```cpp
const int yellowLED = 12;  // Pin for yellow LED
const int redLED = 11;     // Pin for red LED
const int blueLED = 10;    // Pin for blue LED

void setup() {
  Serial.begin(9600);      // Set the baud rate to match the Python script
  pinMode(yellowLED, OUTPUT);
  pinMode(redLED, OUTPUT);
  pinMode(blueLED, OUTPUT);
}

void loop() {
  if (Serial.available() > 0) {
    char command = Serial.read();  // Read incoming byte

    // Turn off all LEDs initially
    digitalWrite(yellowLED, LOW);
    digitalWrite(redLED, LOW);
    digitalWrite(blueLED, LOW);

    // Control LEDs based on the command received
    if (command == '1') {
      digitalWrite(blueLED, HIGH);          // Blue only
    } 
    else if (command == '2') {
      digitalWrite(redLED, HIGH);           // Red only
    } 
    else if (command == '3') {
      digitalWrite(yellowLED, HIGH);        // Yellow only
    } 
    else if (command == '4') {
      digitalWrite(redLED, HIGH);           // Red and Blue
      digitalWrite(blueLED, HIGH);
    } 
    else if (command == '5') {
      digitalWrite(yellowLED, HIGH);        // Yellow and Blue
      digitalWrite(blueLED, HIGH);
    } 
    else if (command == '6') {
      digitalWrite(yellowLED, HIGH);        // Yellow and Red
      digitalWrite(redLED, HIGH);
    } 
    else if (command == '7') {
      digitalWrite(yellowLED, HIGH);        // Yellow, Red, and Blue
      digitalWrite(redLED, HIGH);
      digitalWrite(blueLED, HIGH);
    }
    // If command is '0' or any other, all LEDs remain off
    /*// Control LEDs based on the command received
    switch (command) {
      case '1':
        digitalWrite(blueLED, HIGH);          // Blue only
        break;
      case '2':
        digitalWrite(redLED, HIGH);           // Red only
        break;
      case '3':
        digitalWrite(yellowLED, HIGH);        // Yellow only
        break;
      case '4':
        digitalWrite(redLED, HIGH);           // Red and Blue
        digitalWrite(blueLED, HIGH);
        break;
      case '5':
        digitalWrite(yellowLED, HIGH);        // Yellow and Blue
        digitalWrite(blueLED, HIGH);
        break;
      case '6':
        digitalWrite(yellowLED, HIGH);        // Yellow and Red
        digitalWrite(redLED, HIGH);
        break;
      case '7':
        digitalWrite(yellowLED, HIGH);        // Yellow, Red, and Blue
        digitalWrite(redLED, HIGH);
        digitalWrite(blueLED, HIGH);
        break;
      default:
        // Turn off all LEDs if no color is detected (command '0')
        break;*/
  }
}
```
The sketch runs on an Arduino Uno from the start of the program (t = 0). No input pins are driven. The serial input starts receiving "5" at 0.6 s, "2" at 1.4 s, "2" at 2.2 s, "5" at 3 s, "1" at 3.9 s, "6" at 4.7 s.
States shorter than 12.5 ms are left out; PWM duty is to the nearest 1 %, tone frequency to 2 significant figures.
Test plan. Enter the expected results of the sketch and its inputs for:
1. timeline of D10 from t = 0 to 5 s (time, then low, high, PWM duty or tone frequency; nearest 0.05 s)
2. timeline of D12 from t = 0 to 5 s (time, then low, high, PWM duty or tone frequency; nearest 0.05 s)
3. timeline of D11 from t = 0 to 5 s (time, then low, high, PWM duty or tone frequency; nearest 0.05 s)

0 s low; 0.6 s high; 1.4 s low; 3 s high; 4.7 s low
0 s low; 0.6 s high; 1.4 s low; 3 s high; 3.9 s low; 4.7 s high
0 s low; 1.4 s high; 3 s low; 4.7 s high
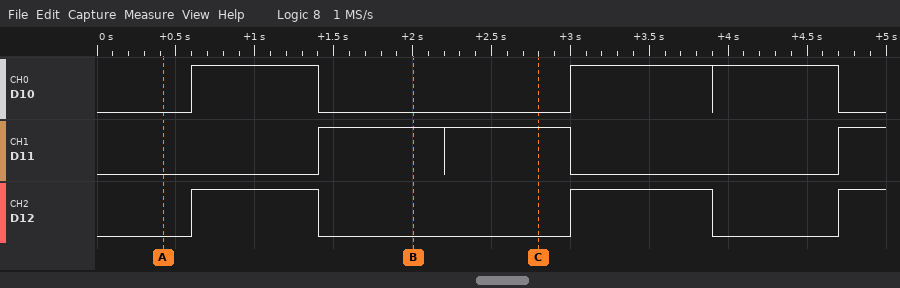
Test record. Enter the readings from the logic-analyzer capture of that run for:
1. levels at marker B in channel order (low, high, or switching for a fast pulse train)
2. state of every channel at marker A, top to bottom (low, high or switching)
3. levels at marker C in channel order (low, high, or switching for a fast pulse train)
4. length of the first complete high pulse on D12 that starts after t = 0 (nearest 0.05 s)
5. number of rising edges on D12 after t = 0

D10 low, D11 high, D12 low
D10 low, D11 low, D12 low
D10 low, D11 high, D12 low
0.80 s
3
